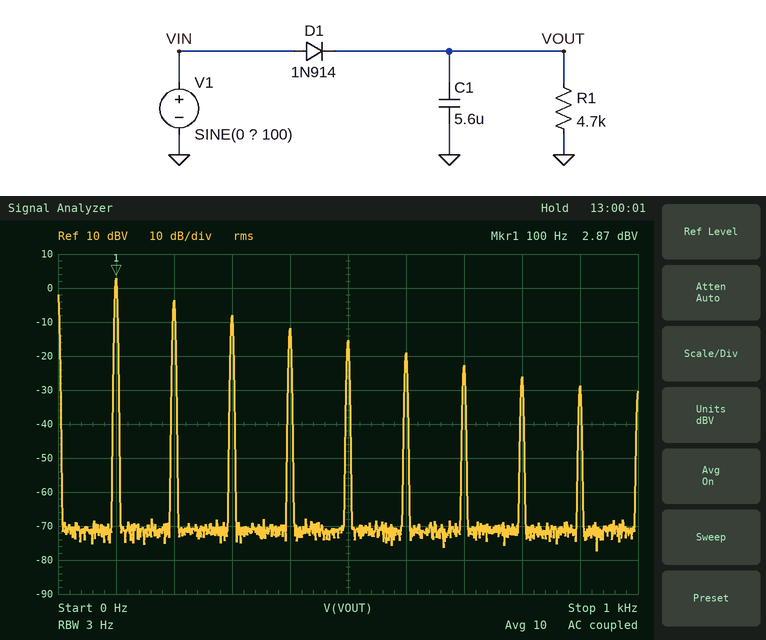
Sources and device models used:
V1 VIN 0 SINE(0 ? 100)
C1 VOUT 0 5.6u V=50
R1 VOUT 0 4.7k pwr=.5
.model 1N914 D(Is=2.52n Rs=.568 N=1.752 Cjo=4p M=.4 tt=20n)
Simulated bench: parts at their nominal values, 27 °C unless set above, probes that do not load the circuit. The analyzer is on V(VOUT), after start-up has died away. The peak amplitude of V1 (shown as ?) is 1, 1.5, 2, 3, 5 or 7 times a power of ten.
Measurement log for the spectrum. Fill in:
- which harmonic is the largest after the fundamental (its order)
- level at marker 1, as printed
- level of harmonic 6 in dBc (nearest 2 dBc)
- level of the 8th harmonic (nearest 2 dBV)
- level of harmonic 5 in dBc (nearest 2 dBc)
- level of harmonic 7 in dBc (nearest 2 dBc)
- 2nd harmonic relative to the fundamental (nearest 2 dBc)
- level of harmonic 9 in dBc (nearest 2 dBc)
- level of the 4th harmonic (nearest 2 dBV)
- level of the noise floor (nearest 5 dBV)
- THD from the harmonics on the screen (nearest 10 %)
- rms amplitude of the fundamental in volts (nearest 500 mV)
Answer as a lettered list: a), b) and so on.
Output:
a) 2
b) 2.87 dBV
c) -22 dBc
d) -26 dBV
e) -18 dBc
f) -26 dBc
g) -6 dBc
h) -32 dBc
i) -12 dBV
j) -70 dBV
k) 60 %
l) 1.5 V
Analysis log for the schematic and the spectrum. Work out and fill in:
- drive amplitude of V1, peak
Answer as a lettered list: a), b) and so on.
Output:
a) 20 V
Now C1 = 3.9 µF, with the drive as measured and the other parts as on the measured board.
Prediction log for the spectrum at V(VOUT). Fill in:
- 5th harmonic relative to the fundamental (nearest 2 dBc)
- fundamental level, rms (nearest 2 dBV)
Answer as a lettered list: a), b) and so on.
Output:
a) -20 dBc
b) 6 dBV
